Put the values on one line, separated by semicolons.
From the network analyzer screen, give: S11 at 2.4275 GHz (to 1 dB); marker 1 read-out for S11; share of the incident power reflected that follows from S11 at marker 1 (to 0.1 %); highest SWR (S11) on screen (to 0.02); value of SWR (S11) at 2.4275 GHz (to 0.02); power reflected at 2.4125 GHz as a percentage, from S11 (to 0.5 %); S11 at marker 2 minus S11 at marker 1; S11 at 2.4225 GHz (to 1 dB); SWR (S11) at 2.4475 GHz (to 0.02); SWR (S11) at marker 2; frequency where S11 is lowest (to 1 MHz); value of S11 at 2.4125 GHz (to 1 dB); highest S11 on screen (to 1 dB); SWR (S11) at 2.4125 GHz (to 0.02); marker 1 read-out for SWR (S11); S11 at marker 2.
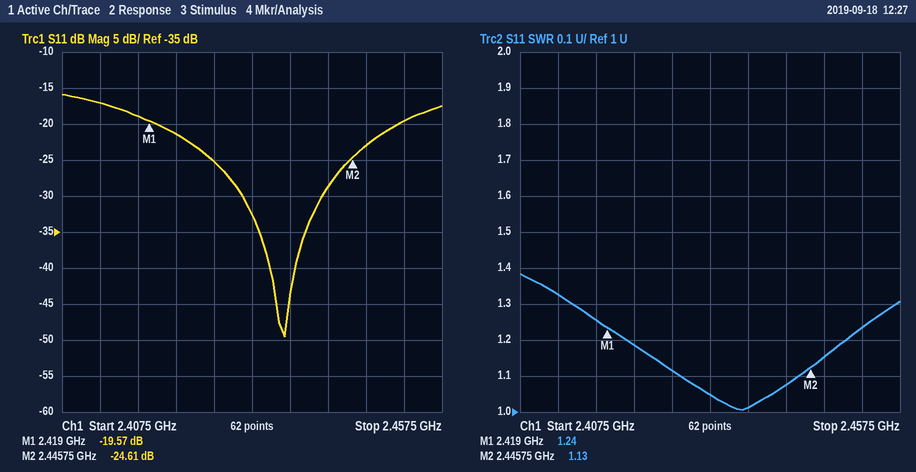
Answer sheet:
-25 dB; -19.57 dB; 1.1 %; 1.38; 1.12; 2.0 %; -5.04 dB; -21 dB; 1.16; 1.13; 2.437 GHz; -17 dB; -16 dB; 1.32; 1.24; -24.61 dB
